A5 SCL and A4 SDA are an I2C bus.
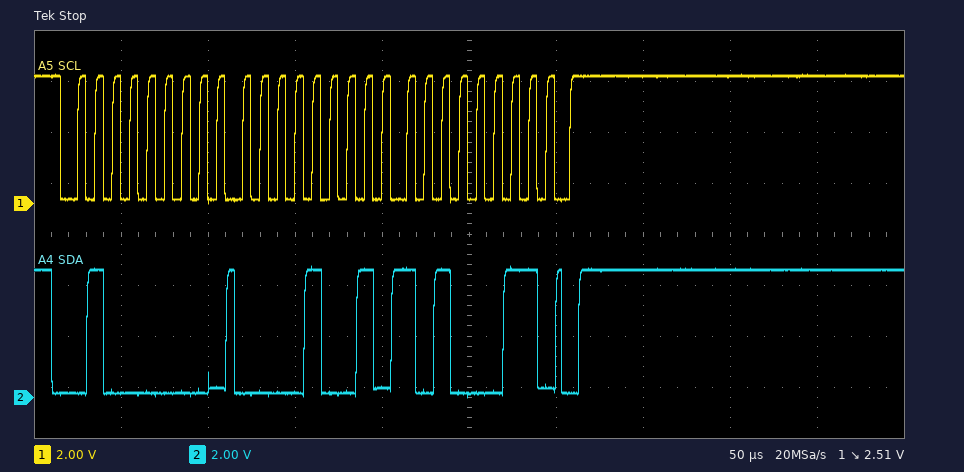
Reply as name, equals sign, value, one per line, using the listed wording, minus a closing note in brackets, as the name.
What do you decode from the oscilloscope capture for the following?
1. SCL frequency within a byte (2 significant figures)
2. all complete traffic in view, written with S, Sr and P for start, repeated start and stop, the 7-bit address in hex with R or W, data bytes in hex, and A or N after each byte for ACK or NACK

SCL frequency within a byte = 100 kHz
all complete traffic in view, written with S, Sr and P for start, repeated start and stop, the 7-bit address in hex with R or W, data bytes in hex, and A or N after each byte for ACK or NACK = S 20W A 09 A A3 A P
